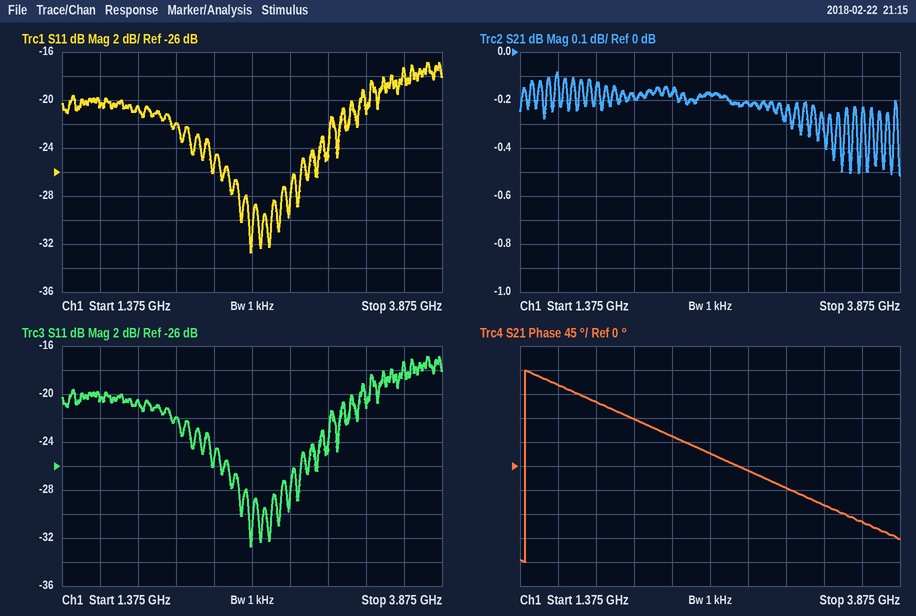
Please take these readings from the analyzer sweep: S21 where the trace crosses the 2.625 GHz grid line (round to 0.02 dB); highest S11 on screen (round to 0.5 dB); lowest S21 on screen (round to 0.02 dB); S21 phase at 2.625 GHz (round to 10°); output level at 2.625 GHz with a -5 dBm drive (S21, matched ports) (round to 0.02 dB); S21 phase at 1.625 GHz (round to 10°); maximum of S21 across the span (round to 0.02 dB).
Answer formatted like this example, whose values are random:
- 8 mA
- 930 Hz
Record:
- -0.18 dB
- -17.0 dB
- -0.52 dB
- 20°
- -5.18 dBm
- 150°
- -0.08 dB
